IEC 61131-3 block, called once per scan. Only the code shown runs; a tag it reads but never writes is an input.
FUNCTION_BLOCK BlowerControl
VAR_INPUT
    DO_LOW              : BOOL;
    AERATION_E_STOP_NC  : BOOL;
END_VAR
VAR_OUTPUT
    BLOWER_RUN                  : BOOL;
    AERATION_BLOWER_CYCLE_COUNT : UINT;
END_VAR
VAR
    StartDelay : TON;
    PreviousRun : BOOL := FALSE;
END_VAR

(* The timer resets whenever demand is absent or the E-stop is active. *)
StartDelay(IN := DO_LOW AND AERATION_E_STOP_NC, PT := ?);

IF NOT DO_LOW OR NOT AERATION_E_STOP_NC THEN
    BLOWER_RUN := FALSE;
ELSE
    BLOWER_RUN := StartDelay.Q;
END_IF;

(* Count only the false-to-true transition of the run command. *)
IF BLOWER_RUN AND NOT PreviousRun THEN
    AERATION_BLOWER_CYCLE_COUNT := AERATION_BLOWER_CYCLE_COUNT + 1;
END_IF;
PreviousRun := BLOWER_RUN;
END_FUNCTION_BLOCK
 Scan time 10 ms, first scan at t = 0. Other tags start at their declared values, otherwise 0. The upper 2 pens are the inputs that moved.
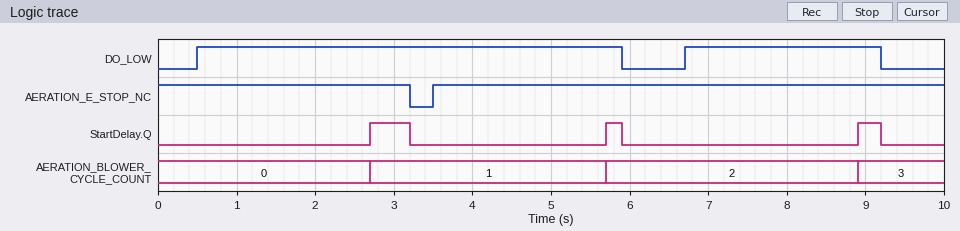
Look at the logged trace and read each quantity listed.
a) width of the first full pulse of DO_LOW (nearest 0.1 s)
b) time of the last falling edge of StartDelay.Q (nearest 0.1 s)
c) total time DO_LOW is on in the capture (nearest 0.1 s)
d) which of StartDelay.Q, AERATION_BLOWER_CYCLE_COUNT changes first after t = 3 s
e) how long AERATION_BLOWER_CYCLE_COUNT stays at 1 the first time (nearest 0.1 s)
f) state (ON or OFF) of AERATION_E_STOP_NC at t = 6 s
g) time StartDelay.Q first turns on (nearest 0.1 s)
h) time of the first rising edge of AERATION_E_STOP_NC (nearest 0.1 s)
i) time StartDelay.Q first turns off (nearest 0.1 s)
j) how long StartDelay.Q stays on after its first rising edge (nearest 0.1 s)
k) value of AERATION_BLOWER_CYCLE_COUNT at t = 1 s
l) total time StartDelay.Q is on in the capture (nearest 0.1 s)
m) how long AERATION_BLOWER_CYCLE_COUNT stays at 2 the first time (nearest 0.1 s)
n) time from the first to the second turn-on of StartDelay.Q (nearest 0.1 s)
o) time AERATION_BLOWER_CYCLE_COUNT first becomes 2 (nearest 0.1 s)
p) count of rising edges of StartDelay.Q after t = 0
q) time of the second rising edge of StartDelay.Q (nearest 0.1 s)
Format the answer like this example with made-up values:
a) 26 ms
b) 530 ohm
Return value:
a) 5.4 s
b) 9.2 s
c) 7.9 s
d) StartDelay.Q
e) 3.0 s
f) ON
g) 2.7 s
h) 3.5 s
i) 3.2 s
j) 0.5 s
k) 0
l) 1.0 s
m) 3.2 s
n) 3.0 s
o) 5.7 s
p) 3
q) 5.7 s
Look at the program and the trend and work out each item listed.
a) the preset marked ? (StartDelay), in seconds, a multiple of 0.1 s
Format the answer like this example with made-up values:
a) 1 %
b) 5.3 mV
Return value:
a) 2.2 s
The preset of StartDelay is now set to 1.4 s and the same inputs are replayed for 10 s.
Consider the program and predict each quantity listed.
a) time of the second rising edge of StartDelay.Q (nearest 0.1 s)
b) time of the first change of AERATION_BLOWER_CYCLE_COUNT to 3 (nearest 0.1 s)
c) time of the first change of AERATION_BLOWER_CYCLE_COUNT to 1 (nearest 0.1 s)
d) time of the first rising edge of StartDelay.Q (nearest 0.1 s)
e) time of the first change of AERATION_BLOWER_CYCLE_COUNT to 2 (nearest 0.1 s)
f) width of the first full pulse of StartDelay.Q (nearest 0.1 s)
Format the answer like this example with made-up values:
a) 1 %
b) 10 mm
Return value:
a) 4.9 s
b) 8.1 s
c) 1.9 s
d) 1.9 s
e) 4.9 s
f) 1.3 s
